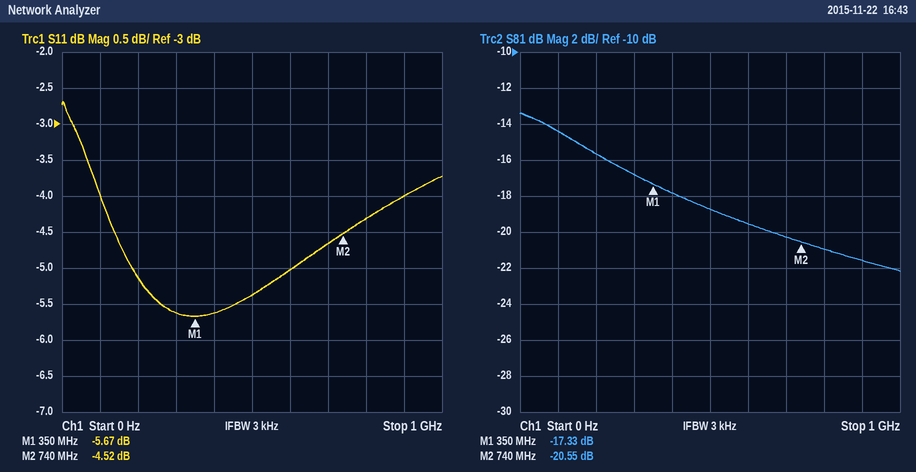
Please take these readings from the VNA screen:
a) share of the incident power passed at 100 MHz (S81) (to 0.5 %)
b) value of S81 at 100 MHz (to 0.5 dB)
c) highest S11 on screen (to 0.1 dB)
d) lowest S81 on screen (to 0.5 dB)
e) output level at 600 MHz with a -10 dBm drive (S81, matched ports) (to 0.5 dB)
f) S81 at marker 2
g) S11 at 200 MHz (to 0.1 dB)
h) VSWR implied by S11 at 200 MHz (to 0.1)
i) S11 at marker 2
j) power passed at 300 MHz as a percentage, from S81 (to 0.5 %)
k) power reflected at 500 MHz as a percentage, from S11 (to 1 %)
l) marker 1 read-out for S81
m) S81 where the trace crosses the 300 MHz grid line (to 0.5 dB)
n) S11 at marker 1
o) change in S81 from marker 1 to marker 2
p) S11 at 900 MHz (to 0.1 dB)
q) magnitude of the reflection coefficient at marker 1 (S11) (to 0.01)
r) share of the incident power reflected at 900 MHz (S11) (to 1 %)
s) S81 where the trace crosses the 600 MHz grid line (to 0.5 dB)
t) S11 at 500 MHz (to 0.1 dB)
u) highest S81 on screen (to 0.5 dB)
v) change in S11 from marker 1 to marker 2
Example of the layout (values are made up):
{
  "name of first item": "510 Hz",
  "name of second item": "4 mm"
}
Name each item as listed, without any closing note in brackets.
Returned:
{
  "share of the incident power passed at 100 MHz (S81)": "3.5 %",
  "value of S81 at 100 MHz": "-14.5 dB",
  "highest S11 on screen": "-2.7 dB",
  "lowest S81 on screen": "-22.0 dB",
  "output level at 600 MHz with a -10 dBm drive (S81, matched ports)": "-29.5 dBm",
  "S81 at marker 2": "-20.55 dB",
  "S11 at 200 MHz": "-5.1 dB",
  "VSWR implied by S11 at 200 MHz": "3.5",
  "S11 at marker 2": "-4.52 dB",
  "power passed at 300 MHz as a percentage, from S81": "2.0 %",
  "power reflected at 500 MHz as a percentage, from S11": "29 %",
  "marker 1 read-out for S81": "-17.33 dB",
  "S81 where the trace crosses the 300 MHz grid line": "-17.0 dB",
  "S11 at marker 1": "-5.67 dB",
  "change in S81 from marker 1 to marker 2": "-3.22 dB",
  "S11 at 900 MHz": "-4.0 dB",
  "magnitude of the reflection coefficient at marker 1 (S11)": "0.52",
  "share of the incident power reflected at 900 MHz (S11)": "40 %",
  "S81 where the trace crosses the 600 MHz grid line": "-19.5 dB",
  "S11 at 500 MHz": "-5.4 dB",
  "highest S81 on screen": "-13.5 dB",
  "change in S11 from marker 1 to marker 2": "1.15 dB"
}
